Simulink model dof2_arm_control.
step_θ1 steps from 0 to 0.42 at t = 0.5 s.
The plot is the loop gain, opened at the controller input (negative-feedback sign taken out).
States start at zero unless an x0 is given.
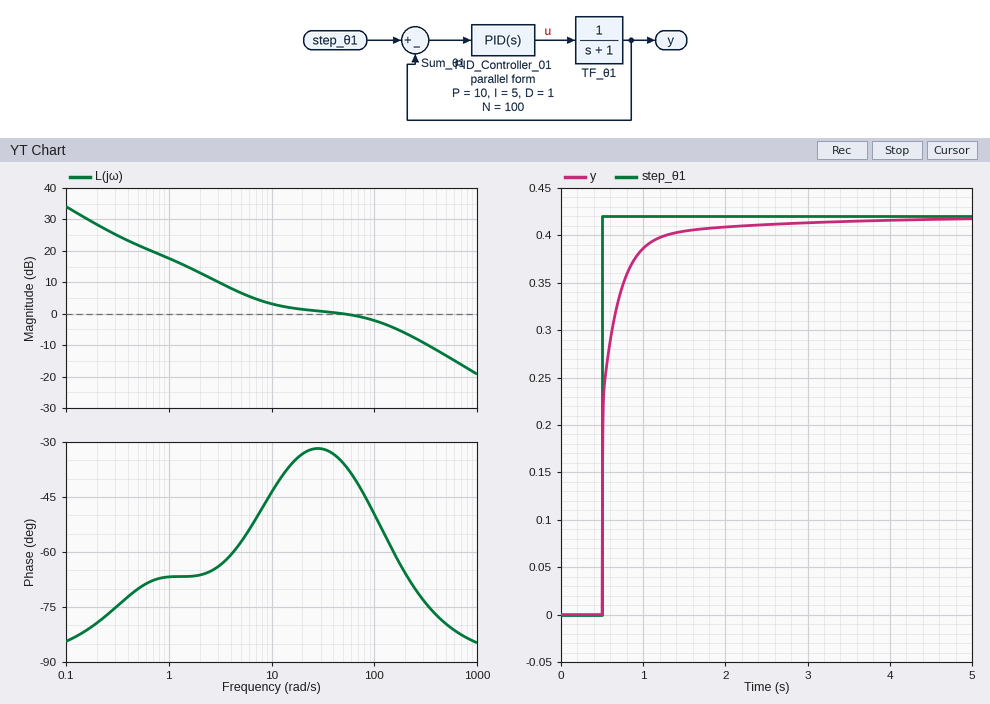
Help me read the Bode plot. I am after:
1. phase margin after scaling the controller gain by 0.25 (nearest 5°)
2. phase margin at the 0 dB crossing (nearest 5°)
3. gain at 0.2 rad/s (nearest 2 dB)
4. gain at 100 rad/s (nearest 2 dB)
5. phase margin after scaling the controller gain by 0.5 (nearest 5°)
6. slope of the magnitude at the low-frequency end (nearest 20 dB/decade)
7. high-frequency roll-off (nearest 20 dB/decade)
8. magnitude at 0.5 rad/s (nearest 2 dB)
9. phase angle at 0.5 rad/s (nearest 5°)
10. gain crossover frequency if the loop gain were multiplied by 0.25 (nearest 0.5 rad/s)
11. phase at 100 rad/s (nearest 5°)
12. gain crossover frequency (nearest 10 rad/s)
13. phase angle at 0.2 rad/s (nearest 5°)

115°
145°
28 dB
-2 dB
125°
-20 dB/decade
-20 dB/decade
22 dB
-70°
2.5 rad/s
-50°
50 rad/s
-80°
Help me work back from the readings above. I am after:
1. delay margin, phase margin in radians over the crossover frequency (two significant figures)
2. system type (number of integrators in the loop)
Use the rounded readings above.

0.051 s
1
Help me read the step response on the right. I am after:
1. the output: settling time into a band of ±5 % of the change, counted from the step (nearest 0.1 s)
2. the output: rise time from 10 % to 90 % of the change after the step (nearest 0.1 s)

0.7 s
0.4 s
